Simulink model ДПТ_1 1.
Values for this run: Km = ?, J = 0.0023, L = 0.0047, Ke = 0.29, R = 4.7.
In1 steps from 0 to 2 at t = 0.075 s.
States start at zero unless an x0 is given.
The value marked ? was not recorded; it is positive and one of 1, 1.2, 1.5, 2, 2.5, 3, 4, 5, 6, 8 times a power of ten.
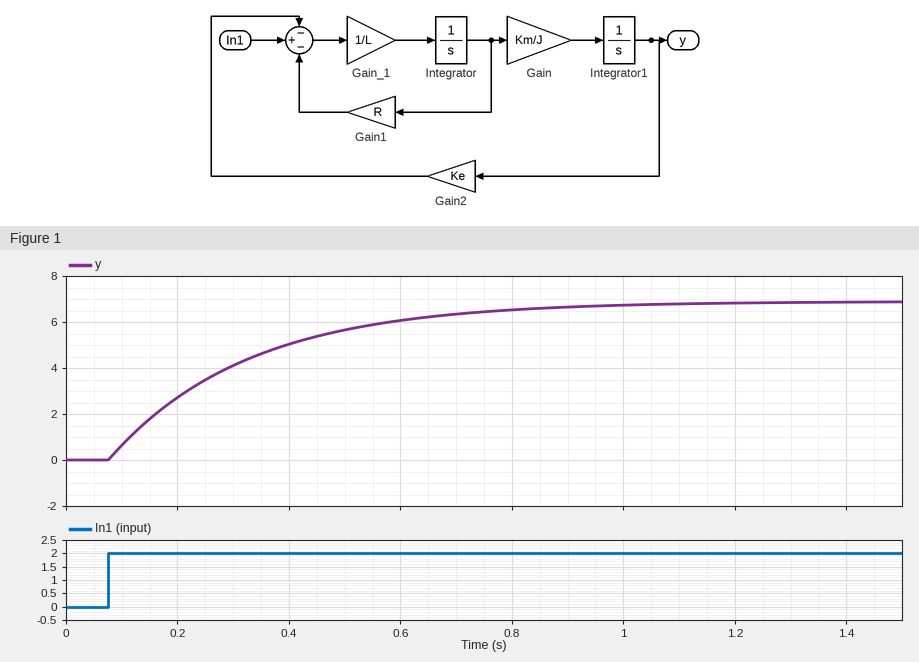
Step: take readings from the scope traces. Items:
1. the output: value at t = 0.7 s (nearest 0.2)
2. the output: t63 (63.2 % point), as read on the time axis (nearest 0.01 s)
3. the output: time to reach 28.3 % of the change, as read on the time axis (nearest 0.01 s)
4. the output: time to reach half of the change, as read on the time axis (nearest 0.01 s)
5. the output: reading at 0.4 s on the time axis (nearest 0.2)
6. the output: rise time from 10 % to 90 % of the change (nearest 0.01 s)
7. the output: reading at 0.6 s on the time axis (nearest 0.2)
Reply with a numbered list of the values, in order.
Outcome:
1. 6.4
2. 0.32 s
3. 0.16 s
4. 0.25 s
5. 5.0
6. 0.54 s
7. 6.0
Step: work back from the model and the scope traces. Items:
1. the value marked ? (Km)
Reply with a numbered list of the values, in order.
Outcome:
1. 0.15
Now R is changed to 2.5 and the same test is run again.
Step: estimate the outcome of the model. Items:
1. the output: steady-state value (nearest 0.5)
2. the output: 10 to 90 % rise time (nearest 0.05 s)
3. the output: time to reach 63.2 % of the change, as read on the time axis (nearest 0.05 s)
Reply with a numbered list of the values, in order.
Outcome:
1. 7.0
2. 0.30 s
3. 0.20 s
